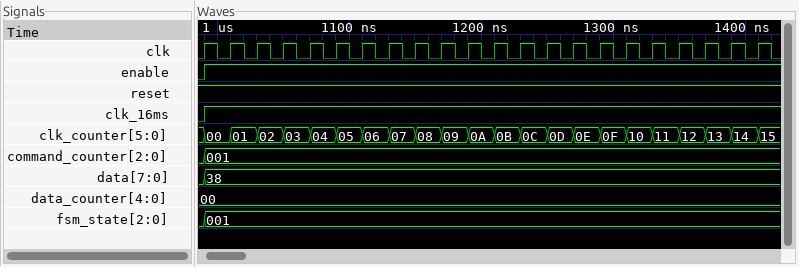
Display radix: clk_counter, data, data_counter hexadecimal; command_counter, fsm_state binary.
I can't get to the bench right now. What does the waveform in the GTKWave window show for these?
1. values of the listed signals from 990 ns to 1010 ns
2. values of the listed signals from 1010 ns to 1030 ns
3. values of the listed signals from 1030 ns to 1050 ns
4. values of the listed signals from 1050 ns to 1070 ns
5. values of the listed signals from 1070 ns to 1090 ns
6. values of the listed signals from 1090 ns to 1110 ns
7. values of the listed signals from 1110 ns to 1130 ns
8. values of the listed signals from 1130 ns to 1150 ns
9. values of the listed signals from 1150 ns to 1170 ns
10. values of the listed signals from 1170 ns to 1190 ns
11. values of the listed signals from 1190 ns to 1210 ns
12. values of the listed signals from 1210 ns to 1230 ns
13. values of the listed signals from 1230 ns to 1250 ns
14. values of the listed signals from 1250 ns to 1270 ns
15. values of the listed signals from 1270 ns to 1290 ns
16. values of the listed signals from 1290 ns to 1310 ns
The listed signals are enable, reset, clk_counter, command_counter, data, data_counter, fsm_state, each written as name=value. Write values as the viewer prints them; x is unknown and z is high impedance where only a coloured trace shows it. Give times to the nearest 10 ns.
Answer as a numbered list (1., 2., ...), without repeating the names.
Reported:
1. enable=1, reset=1, clk_counter=00, command_counter=001, data=38, data_counter=00, fsm_state=001
2. enable=1, reset=1, clk_counter=01, command_counter=001, data=38, data_counter=00, fsm_state=001
3. enable=1, reset=1, clk_counter=02, command_counter=001, data=38, data_counter=00, fsm_state=001
4. enable=1, reset=1, clk_counter=03, command_counter=001, data=38, data_counter=00, fsm_state=001
5. enable=1, reset=1, clk_counter=04, command_counter=001, data=38, data_counter=00, fsm_state=001
6. enable=1, reset=1, clk_counter=05, command_counter=001, data=38, data_counter=00, fsm_state=001
7. enable=1, reset=1, clk_counter=06, command_counter=001, data=38, data_counter=00, fsm_state=001
8. enable=1, reset=1, clk_counter=07, command_counter=001, data=38, data_counter=00, fsm_state=001
9. enable=1, reset=1, clk_counter=08, command_counter=001, data=38, data_counter=00, fsm_state=001
10. enable=1, reset=1, clk_counter=09, command_counter=001, data=38, data_counter=00, fsm_state=001
11. enable=1, reset=1, clk_counter=0A, command_counter=001, data=38, data_counter=00, fsm_state=001
12. enable=1, reset=1, clk_counter=0B, command_counter=001, data=38, data_counter=00, fsm_state=001
13. enable=1, reset=1, clk_counter=0C, command_counter=001, data=38, data_counter=00, fsm_state=001
14. enable=1, reset=1, clk_counter=0D, command_counter=001, data=38, data_counter=00, fsm_state=001
15. enable=1, reset=1, clk_counter=0E, command_counter=001, data=38, data_counter=00, fsm_state=001
16. enable=1, reset=1, clk_counter=0F, command_counter=001, data=38, data_counter=00, fsm_state=001
